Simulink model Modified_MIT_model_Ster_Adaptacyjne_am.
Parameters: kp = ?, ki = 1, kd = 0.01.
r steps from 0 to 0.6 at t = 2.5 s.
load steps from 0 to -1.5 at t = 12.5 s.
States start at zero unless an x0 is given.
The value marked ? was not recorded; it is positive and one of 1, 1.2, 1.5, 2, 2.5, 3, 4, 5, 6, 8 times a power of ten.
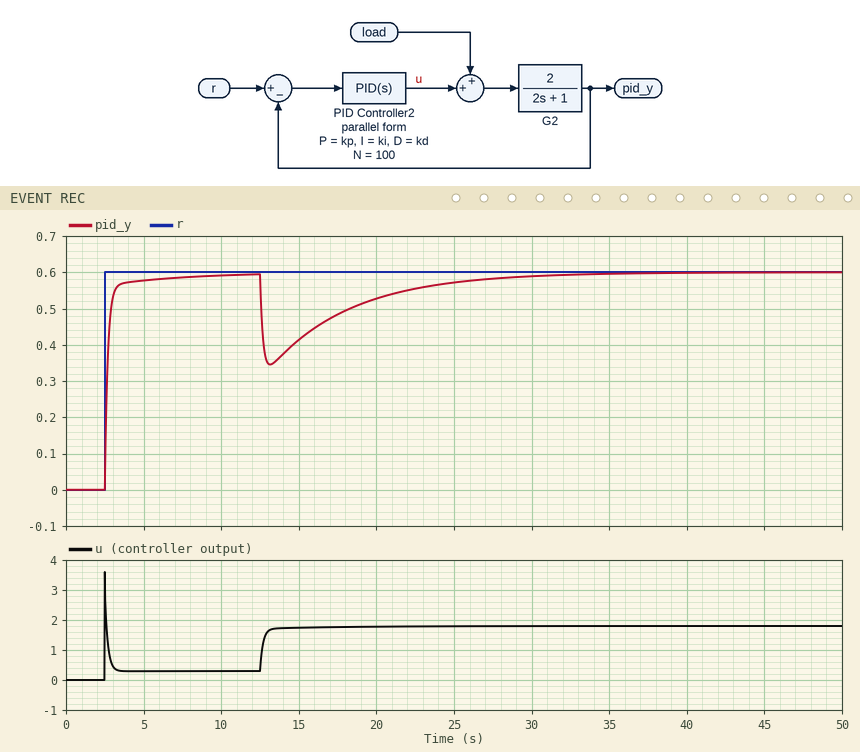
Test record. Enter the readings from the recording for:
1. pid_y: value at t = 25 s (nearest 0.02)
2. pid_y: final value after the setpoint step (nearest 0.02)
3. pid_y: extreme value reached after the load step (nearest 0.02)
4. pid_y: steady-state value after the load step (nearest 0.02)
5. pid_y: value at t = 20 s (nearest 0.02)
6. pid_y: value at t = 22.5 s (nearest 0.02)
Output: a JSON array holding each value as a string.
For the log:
["0.58", "0.60", "0.34", "0.60", "0.52", "0.56"]
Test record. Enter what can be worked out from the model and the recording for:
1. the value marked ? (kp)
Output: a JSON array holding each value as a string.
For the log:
["5"]
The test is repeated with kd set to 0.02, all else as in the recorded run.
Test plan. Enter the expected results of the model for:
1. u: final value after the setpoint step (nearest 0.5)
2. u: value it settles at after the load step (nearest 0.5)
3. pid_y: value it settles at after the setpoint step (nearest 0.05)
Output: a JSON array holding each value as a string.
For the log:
["0.5", "2.0", "0.60"]
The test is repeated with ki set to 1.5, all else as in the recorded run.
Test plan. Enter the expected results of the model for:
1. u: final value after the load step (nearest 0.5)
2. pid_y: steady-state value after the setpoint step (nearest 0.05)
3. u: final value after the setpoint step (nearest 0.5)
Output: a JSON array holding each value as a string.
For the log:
["2.0", "0.60", "0.5"]
